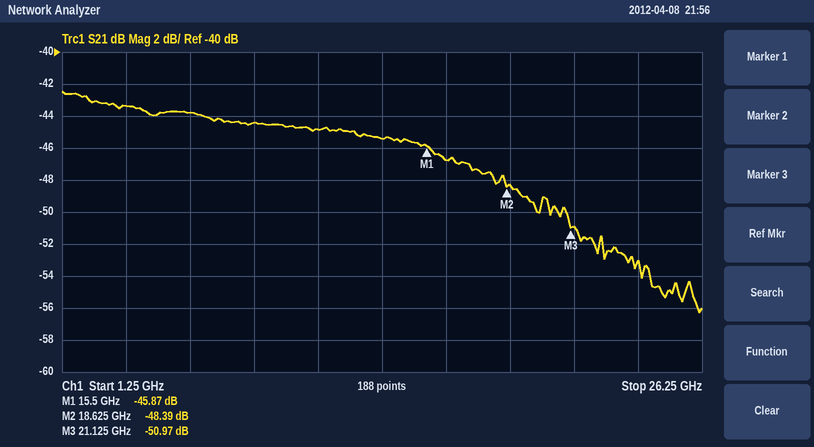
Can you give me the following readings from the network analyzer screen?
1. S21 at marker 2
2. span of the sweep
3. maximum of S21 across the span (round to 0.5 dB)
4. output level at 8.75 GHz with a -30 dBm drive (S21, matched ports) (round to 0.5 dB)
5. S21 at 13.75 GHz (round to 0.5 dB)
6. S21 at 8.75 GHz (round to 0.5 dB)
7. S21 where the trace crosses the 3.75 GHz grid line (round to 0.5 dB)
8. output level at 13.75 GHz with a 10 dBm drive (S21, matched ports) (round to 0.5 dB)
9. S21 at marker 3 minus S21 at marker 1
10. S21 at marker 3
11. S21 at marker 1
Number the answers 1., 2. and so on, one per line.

1. -48.39 dB
2. 25 GHz
3. -42.5 dB
4. -74.5 dBm
5. -45.5 dB
6. -44.5 dB
7. -43.5 dB
8. -35.5 dBm
9. -5.10 dB
10. -50.97 dB
11. -45.87 dB
